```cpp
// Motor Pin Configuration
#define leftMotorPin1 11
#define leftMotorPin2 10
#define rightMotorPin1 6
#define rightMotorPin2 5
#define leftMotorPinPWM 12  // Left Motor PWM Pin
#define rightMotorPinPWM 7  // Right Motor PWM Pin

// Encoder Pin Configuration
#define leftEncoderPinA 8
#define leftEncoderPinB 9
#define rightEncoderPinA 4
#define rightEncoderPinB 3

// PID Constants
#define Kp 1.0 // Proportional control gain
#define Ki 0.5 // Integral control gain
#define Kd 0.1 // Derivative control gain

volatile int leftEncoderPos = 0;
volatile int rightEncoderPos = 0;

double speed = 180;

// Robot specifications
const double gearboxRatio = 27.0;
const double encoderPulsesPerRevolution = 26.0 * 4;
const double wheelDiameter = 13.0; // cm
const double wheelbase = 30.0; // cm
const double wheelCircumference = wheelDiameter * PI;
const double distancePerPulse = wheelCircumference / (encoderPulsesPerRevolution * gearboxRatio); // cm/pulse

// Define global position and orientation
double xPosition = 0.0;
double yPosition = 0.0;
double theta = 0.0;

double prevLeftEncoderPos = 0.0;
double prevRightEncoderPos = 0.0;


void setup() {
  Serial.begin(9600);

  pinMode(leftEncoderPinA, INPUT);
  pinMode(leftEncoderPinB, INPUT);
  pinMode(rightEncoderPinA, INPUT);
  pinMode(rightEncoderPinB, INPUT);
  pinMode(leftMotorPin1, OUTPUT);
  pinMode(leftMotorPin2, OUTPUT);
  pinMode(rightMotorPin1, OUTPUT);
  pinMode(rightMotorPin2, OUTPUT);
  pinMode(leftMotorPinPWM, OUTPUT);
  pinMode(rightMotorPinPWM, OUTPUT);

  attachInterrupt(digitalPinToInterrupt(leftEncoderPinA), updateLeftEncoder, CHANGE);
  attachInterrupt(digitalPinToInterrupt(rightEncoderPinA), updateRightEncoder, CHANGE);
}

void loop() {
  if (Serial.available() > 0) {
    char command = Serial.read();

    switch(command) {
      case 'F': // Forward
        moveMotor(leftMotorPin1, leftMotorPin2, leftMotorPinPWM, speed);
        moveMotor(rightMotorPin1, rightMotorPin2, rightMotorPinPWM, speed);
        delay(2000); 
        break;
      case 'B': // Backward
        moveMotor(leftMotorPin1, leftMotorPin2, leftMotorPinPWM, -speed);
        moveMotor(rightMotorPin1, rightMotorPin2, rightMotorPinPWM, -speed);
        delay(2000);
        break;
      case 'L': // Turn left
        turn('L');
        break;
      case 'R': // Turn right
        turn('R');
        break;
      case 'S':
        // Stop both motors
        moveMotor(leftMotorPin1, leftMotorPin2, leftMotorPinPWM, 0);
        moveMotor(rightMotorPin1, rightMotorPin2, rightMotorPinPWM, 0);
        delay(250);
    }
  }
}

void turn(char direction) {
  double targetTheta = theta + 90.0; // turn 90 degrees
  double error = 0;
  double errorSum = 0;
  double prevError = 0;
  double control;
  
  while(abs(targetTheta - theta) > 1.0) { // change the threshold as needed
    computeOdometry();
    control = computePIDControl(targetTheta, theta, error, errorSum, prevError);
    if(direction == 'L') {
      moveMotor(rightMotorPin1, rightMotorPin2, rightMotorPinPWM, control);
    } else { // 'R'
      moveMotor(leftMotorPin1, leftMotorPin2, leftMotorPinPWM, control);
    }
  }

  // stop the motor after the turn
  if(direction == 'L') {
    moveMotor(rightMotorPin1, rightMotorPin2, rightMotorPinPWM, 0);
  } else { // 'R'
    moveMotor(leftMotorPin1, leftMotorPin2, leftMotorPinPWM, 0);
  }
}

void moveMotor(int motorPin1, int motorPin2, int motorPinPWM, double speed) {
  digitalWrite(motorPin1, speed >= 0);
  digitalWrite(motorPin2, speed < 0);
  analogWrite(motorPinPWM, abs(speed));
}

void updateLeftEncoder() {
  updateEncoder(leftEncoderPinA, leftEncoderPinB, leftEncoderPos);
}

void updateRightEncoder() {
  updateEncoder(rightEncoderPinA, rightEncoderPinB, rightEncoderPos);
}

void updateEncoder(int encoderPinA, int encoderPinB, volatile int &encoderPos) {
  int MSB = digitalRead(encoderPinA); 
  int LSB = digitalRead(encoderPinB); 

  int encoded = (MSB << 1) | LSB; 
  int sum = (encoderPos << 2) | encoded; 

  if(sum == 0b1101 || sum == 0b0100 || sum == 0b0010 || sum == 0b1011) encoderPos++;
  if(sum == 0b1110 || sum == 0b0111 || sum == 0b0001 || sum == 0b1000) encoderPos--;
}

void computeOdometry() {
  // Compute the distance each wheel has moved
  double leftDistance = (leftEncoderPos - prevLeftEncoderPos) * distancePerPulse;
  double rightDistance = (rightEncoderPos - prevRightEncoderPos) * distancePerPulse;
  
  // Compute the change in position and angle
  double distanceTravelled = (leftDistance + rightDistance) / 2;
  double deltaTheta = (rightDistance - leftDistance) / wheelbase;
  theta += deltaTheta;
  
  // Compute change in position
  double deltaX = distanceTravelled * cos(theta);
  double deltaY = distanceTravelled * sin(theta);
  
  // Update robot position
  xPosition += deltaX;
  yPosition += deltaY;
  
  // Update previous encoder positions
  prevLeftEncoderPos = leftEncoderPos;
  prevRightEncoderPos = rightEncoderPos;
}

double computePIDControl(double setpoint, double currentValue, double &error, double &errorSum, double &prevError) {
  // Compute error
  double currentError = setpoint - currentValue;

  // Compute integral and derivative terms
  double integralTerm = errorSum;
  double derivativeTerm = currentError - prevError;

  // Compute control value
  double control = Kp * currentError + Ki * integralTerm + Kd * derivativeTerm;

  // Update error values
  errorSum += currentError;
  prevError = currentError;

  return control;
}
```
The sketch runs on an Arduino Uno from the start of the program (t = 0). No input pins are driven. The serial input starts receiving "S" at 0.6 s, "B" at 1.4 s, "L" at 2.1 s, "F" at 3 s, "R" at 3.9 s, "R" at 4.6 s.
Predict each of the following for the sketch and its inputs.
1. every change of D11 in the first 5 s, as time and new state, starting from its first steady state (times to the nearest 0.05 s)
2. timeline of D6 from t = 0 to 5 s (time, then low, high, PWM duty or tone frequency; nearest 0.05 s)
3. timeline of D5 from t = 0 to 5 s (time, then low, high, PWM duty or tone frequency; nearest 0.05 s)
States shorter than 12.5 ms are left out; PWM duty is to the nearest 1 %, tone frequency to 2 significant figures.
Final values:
0 s low; 0.6 s high; 1.4 s low
0 s low; 0.6 s high; 1.4 s low; 3.4 s high
0 s low; 1.4 s high; 3.4 s low
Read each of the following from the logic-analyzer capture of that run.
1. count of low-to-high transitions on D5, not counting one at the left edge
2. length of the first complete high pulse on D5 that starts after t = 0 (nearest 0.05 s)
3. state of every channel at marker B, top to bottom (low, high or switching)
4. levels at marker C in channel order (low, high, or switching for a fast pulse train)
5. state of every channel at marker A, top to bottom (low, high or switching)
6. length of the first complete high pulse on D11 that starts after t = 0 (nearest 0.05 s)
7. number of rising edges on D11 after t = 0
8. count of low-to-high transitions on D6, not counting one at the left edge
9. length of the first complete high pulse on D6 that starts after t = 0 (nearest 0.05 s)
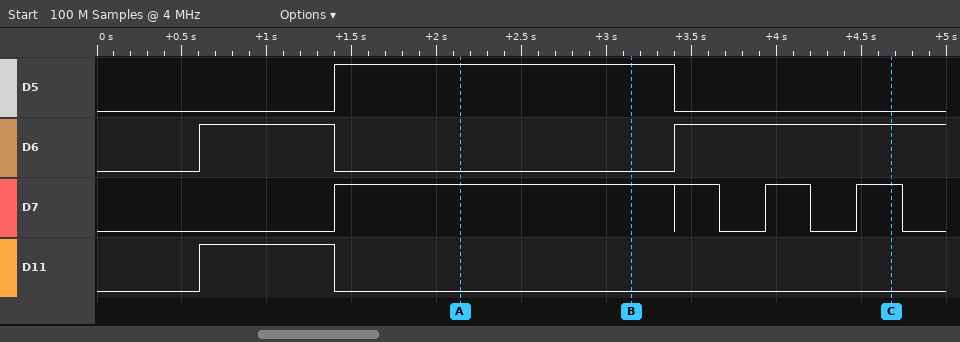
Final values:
1
2.00 s
D5 high, D6 low, D7 high, D11 low
D5 low, D6 high, D7 high, D11 low
D5 high, D6 low, D7 high, D11 low
0.80 s
1
2
0.80 s
